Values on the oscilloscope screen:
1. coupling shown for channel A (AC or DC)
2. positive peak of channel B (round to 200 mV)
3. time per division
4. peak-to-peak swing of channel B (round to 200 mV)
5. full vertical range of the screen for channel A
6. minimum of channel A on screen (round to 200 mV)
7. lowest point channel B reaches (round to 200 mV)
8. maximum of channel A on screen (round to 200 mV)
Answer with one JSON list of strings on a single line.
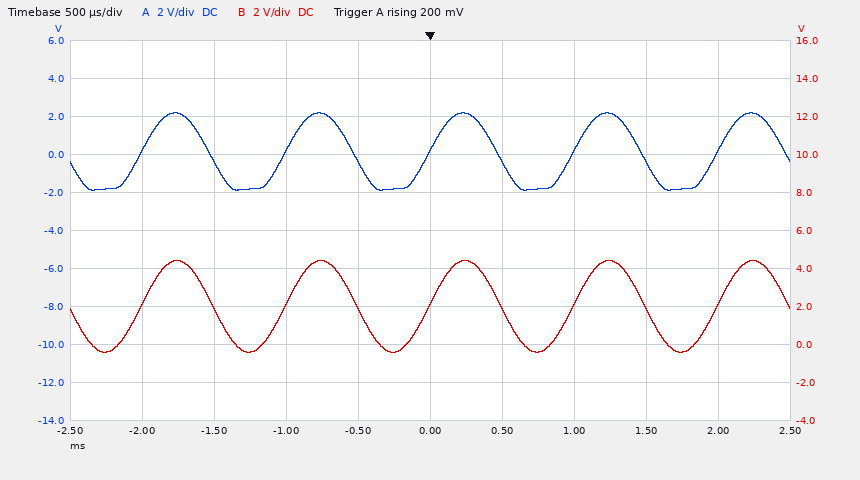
["DC", "4.4 V", "500 µs", "4.8 V", "20 V", "-1.8 V", "-400 mV", "2.2 V"]
